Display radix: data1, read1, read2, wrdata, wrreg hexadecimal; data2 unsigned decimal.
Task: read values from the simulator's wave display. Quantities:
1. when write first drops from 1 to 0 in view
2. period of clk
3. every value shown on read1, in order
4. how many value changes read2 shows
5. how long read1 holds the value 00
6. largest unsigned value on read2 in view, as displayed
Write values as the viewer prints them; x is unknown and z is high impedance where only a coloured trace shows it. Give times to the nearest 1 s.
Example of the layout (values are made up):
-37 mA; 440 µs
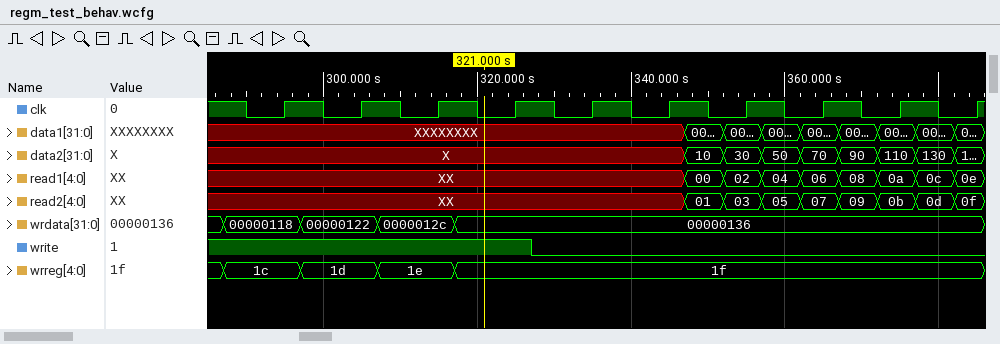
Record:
327 s; 10 s; XX, 00, 02, 04, 06, 08, 0a, 0c, 0e; 8; 5 s; 0f
